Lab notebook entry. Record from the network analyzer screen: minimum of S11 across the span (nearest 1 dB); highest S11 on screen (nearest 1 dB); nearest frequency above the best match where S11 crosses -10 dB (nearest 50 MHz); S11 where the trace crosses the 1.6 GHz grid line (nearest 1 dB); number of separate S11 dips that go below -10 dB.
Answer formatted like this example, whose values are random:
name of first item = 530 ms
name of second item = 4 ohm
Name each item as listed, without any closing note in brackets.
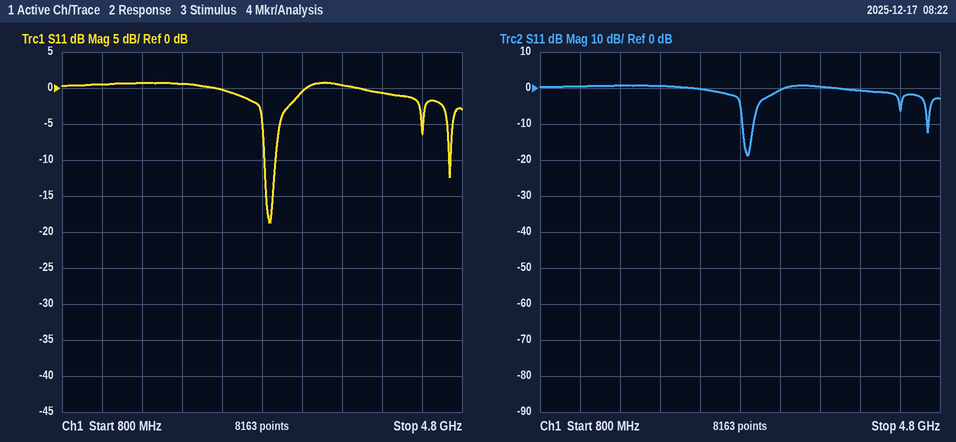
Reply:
minimum of S11 across the span = -19 dB
highest S11 on screen = 1 dB
nearest frequency above the best match where S11 crosses -10 dB = 2.95 GHz
S11 where the trace crosses the 1.6 GHz grid line = 1 dB
number of separate S11 dips that go below -10 dB = 2
